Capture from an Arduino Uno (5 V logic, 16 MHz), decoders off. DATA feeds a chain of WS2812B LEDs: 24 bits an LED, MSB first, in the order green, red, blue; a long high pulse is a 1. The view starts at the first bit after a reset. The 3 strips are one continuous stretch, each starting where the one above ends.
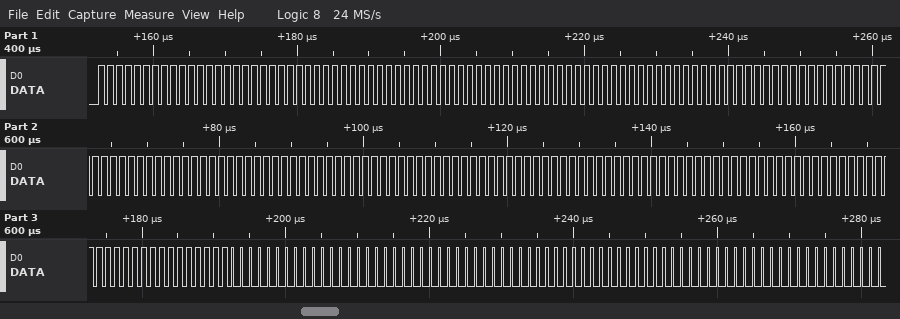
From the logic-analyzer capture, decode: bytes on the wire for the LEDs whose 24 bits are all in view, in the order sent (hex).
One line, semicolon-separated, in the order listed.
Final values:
FF FF FF FF FF FF FF FF FF FF FF FF FF FF FF FF FF FF FF FF FF FF FF FF 00 00 00 00 00 00 00 00 00
